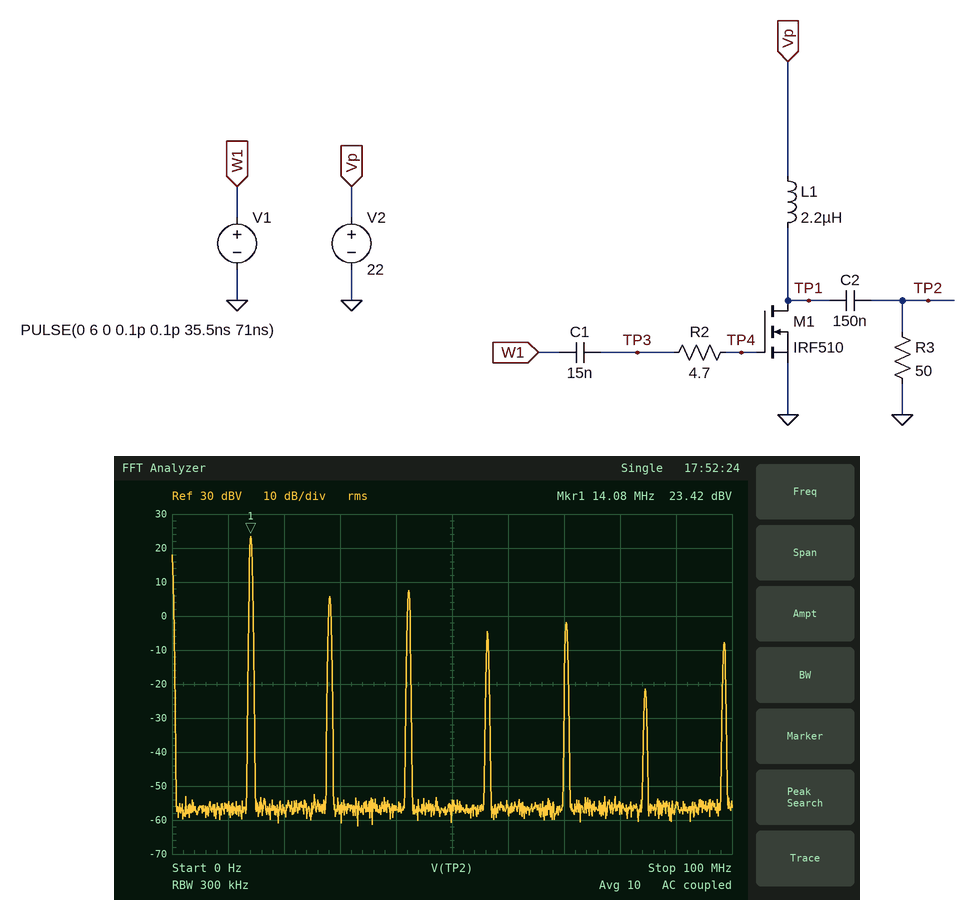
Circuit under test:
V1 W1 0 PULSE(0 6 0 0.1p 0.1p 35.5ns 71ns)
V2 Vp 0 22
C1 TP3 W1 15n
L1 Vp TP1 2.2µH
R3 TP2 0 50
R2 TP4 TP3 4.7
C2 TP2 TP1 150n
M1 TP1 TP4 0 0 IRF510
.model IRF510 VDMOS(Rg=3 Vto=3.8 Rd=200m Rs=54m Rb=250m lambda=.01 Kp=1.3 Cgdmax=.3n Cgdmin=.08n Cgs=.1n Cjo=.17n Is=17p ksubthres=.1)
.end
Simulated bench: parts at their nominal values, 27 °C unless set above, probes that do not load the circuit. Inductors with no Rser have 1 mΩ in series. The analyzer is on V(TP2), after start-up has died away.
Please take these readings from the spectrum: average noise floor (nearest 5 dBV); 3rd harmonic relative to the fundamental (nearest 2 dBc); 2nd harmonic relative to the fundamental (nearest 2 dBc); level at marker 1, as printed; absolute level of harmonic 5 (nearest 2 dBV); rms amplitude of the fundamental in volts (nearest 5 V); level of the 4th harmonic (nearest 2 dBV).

-55 dBV
-16 dBc
-18 dBc
23.42 dBV
-2 dBV
15 V
-4 dBV
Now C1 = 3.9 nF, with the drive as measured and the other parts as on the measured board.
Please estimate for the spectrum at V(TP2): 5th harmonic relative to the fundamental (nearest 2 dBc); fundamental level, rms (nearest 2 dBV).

-24 dBc
22 dBV
